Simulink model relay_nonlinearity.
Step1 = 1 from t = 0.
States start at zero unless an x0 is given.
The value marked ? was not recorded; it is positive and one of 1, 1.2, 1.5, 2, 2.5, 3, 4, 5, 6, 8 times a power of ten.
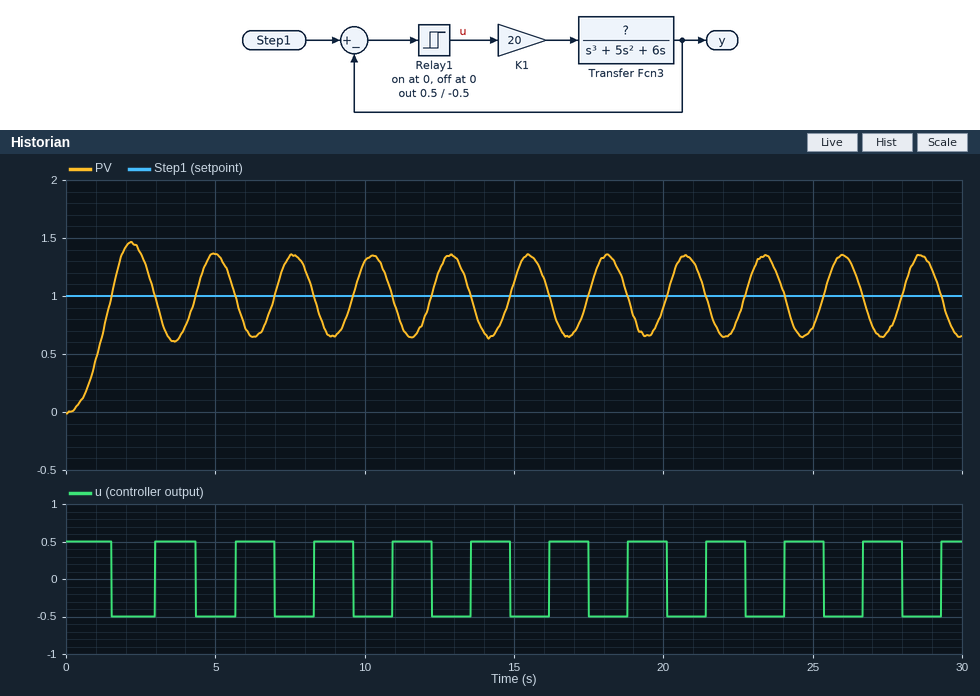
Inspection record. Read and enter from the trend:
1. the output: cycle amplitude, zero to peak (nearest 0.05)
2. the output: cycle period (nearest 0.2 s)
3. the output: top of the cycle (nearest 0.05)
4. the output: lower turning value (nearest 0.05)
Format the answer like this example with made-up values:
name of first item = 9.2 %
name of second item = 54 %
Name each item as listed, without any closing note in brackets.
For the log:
the output: cycle amplitude, zero to peak = 0.35
the output: cycle period = 2.6 s
the output: top of the cycle = 1.35
the output: lower turning value = 0.65
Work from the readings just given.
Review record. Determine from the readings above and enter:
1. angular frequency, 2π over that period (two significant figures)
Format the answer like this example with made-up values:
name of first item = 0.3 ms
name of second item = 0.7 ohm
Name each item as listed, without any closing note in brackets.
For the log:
angular frequency, 2π over that period = 2.4 rad/s
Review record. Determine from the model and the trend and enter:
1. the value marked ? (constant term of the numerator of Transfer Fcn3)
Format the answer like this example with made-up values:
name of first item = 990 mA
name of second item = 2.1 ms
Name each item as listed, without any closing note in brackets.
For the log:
the value marked ? = 0.8
